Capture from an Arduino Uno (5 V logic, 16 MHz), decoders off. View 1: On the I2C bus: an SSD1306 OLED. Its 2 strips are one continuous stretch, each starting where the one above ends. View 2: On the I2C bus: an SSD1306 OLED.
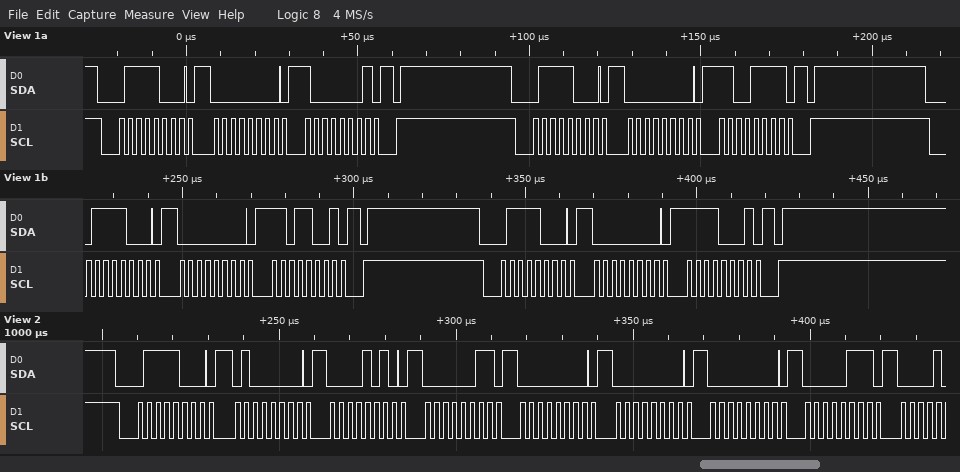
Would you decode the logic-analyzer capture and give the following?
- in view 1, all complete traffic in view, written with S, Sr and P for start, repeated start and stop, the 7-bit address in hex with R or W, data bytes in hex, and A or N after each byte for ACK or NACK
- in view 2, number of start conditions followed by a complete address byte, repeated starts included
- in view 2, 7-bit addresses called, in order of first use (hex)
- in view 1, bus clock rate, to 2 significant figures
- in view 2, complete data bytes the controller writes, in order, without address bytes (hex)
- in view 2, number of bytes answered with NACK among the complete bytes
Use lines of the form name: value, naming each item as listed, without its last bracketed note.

in view 1, all complete traffic in view, written with S, Sr and P for start, repeated start and stop, the 7-bit address in hex with R or W, data bytes in hex, and A or N after each byte for ACK or NACK: S 3CW A 00 A 81 A P S 3CW A 00 A CF A P S 3CW A 00 A D9 A P S 3CW A 00 A F1 A P
in view 2, number of start conditions followed by a complete address byte, repeated starts included: 1
in view 2, 7-bit addresses called, in order of first use: 0x3C
in view 1, bus clock rate, to 2 significant figures: 400 kHz
in view 2, complete data bytes the controller writes, in order, without address bytes: 40 0A 03 00 00 00 07
in view 2, number of bytes answered with NACK among the complete bytes: 0
